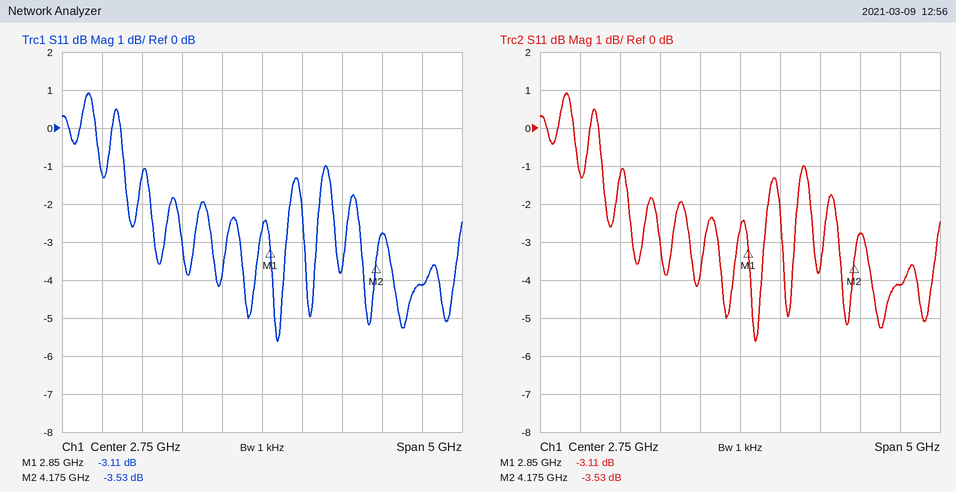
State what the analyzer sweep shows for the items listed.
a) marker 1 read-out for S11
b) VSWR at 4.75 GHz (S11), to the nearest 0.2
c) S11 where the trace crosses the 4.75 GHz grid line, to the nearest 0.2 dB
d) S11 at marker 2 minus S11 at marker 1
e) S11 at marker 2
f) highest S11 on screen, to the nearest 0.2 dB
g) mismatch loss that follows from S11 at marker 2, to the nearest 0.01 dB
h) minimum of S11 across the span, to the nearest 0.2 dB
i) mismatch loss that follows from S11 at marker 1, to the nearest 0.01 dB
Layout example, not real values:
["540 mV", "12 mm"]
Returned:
["-3.11 dB", "4.2", "-4.2 dB", "-0.42 dB", "-3.53 dB", "1.0 dB", "2.55 dB", "-5.6 dB", "2.91 dB"]
